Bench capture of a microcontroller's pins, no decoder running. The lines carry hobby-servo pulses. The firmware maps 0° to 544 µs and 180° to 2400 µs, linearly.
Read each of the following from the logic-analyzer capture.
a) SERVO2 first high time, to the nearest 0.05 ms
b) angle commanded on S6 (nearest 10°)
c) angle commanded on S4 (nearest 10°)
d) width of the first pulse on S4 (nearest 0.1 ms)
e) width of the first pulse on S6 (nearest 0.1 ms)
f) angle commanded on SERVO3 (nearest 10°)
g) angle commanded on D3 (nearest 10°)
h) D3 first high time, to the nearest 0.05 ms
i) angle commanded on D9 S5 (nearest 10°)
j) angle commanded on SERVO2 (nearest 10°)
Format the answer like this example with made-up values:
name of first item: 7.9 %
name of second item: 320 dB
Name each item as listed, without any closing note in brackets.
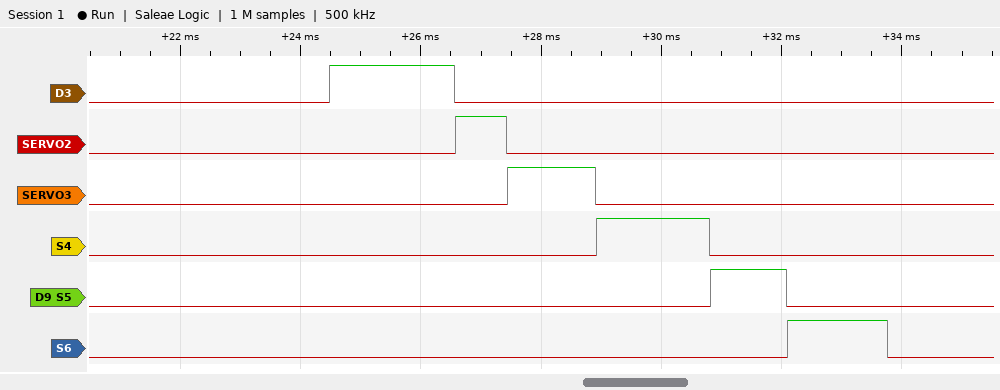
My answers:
SERVO2 first high time, to the nearest 0.05 ms: 0.85 ms
angle commanded on S6: 110°
angle commanded on S4: 130°
width of the first pulse on S4: 1.9 ms
width of the first pulse on S6: 1.7 ms
angle commanded on SERVO3: 90°
angle commanded on D3: 150°
D3 first high time, to the nearest 0.05 ms: 2.10 ms
angle commanded on D9 S5: 70°
angle commanded on SERVO2: 30°
